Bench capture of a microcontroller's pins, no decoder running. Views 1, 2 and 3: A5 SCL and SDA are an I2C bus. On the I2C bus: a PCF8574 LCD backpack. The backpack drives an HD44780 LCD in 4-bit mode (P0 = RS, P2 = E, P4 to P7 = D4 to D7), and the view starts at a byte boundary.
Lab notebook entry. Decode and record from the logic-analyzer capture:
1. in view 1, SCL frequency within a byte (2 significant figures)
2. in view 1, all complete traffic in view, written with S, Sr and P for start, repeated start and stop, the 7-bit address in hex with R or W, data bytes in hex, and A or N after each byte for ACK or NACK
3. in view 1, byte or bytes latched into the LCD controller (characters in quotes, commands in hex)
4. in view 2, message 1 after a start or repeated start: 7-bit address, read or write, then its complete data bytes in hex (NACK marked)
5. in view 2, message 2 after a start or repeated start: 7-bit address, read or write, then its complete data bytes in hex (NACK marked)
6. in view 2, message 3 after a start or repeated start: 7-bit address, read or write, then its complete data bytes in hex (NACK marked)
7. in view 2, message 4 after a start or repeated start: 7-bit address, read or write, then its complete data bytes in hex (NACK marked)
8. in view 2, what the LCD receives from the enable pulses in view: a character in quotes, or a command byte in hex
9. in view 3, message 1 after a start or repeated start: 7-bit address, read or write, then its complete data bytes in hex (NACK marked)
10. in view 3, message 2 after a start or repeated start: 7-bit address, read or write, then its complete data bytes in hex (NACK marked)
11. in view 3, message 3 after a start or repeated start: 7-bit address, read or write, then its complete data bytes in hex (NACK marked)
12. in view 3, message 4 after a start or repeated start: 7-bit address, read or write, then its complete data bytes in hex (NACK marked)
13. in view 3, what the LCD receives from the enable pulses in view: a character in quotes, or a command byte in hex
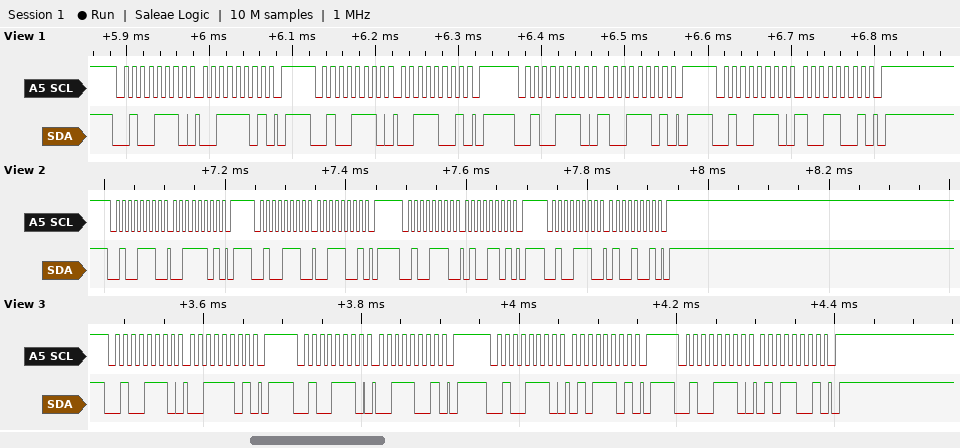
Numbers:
100 kHz
S 27W A 3D A P S 27W A 39 A P S 27W A 9D A P S 27W A 99 A P
'9'
0x27 write: 3D
0x27 write: 39
0x27 write: 4D
0x27 write: 49
'4'
0x27 write: 3D
0x27 write: 39
0x27 write: 5D
0x27 write: 59
'5'
